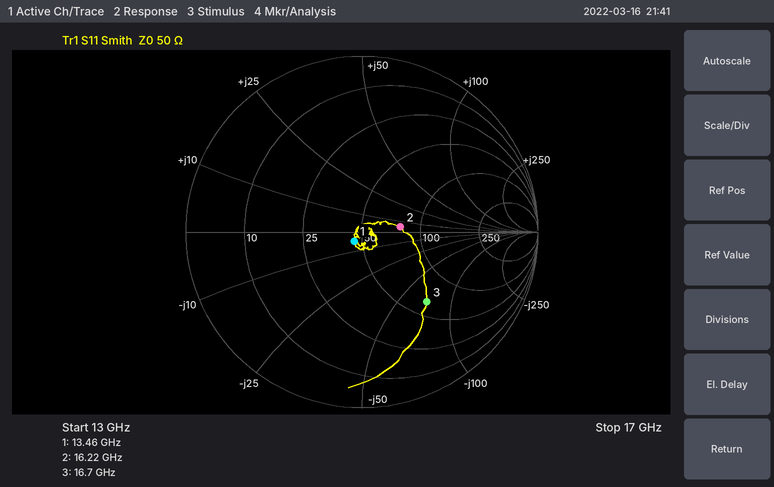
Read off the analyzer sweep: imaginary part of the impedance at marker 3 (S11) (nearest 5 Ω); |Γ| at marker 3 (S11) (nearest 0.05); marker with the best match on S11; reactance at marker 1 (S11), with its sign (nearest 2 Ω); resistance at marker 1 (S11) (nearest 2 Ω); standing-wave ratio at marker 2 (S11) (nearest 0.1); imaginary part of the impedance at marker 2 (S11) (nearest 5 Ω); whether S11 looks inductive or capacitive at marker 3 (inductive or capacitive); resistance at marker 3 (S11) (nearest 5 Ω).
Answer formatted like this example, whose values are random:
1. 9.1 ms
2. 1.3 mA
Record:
1. -70 Ω
2. 0.55
3. marker 1
4. -4 Ω
5. 46 Ω
6. 1.6
7. +5 Ω
8. capacitive
9. 65 Ω
